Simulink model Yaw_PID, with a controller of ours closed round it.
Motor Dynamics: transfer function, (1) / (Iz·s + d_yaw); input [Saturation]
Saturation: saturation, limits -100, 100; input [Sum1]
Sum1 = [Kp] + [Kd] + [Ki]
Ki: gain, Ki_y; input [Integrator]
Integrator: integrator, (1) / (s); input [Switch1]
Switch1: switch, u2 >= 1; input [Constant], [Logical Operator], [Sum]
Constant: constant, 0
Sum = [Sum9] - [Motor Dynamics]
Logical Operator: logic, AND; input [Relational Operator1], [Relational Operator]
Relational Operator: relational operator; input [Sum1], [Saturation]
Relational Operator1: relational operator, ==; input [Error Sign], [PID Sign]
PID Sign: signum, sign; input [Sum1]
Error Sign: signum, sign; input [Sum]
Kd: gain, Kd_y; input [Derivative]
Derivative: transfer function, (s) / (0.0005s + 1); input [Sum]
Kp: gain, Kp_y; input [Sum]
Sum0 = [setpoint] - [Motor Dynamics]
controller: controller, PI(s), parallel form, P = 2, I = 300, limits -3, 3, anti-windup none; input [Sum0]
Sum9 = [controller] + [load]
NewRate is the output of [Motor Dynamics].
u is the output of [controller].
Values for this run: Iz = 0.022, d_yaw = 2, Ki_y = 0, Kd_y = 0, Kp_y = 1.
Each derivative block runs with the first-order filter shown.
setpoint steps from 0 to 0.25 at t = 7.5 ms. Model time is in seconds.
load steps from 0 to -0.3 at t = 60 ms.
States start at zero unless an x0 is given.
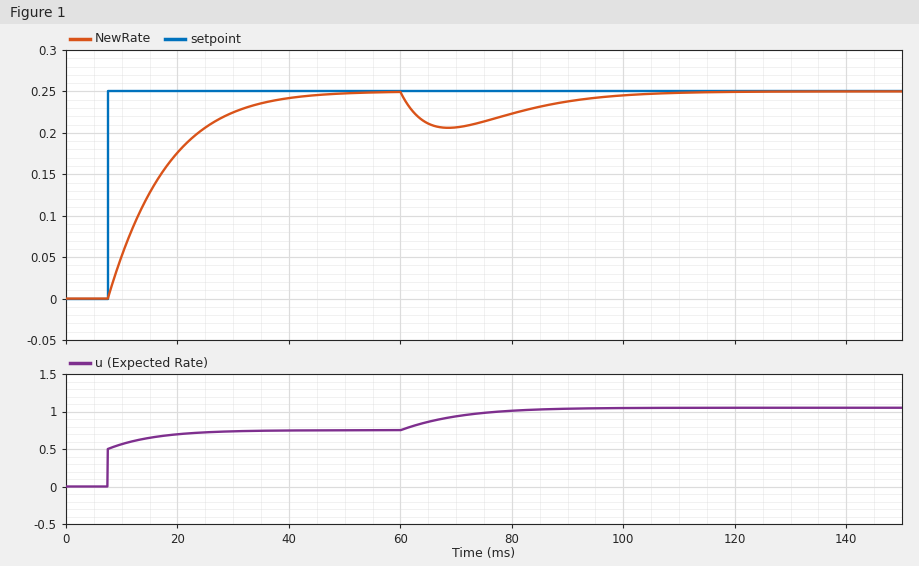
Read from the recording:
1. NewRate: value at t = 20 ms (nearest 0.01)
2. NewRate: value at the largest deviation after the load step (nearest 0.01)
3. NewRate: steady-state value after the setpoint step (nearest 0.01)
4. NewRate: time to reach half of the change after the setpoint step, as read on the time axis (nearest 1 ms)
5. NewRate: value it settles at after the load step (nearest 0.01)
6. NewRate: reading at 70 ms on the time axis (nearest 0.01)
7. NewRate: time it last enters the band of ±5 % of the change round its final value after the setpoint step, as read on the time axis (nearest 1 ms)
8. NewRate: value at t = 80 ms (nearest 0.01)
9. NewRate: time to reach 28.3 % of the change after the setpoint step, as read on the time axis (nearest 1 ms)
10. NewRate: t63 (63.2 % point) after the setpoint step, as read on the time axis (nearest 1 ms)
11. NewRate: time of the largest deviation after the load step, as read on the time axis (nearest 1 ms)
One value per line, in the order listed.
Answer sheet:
0.18
0.21
0.25
15 ms
0.25
0.21
36 ms
0.22
11 ms
18 ms
69 ms
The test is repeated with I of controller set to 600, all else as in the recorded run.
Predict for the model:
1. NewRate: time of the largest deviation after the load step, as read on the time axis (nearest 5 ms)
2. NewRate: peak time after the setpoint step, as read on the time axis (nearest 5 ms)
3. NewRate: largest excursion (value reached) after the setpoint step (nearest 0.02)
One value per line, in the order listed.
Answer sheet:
65 ms
30 ms
0.26
